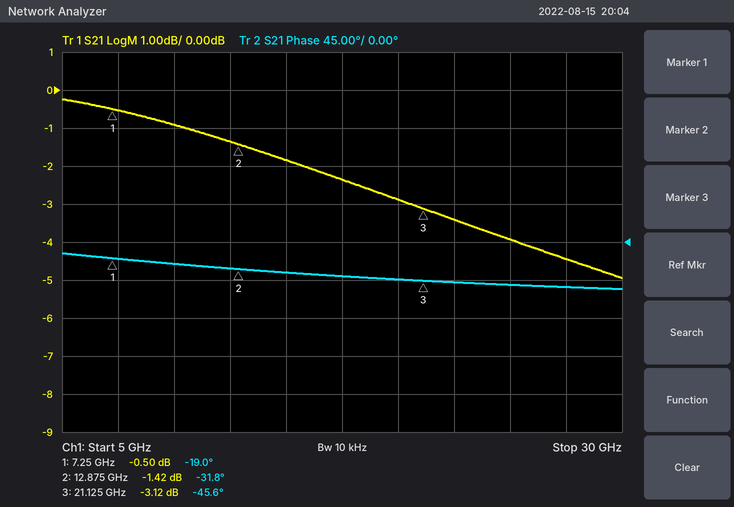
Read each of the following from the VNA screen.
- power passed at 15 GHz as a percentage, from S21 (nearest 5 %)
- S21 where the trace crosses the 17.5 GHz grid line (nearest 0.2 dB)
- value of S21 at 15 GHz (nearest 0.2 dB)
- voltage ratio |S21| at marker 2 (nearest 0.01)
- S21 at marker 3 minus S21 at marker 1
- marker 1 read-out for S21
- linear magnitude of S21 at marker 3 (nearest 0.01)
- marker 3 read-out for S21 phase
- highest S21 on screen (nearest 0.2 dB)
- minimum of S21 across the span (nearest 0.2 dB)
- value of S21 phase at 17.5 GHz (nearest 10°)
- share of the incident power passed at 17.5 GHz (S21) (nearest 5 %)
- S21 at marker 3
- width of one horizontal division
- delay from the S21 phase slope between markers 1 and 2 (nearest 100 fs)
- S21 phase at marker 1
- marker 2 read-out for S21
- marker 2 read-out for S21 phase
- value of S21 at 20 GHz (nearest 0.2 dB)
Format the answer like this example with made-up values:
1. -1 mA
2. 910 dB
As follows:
1. 65 %
2. -2.4 dB
3. -1.8 dB
4. 0.85
5. -2.62 dB
6. -0.50 dB
7. 0.70
8. -45.6°
9. -0.2 dB
10. -5.0 dB
11. -40°
12. 60 %
13. -3.12 dB
14. 2.5 GHz
15. 6.3 ps
16. -19.0°
17. -1.42 dB
18. -31.8°
19. -2.8 dB
